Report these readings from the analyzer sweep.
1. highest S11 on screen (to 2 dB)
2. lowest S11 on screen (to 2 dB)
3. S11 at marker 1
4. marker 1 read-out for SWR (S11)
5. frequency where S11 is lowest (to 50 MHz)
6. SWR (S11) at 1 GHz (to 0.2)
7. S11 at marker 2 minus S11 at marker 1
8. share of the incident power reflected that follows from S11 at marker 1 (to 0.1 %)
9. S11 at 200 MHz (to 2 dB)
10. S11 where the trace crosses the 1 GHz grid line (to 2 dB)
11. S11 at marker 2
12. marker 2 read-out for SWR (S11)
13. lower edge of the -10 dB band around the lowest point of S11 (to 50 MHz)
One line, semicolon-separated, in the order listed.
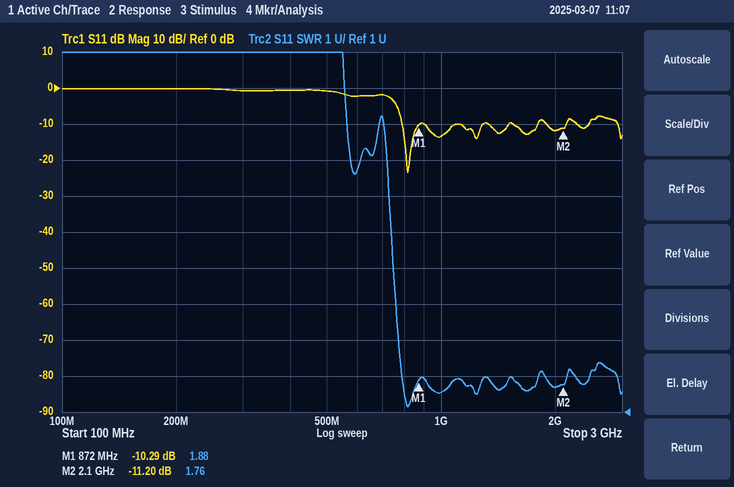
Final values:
0 dB; -24 dB; -10.29 dB; 1.88; 800 MHz; 1.6; -0.91 dB; 9.4 %; 0 dB; -14 dB; -11.20 dB; 1.76; 800 MHz
